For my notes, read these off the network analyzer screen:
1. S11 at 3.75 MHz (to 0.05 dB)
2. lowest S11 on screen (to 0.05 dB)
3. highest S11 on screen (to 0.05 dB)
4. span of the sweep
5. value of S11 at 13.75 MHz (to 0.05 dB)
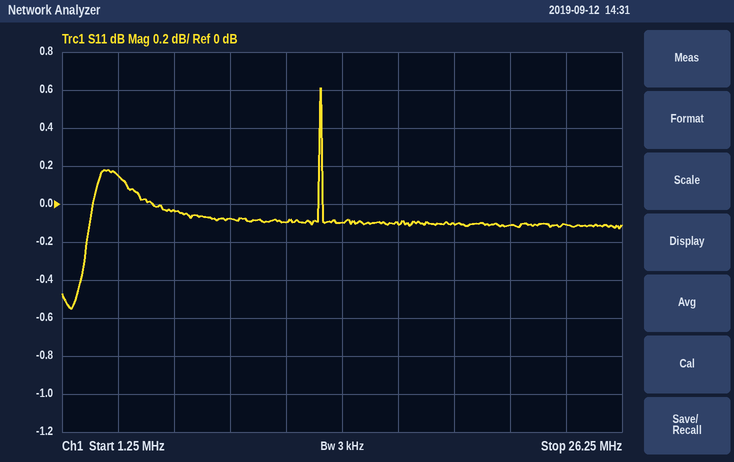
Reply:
0.15 dB
-0.55 dB
0.60 dB
25 MHz
-0.10 dB
